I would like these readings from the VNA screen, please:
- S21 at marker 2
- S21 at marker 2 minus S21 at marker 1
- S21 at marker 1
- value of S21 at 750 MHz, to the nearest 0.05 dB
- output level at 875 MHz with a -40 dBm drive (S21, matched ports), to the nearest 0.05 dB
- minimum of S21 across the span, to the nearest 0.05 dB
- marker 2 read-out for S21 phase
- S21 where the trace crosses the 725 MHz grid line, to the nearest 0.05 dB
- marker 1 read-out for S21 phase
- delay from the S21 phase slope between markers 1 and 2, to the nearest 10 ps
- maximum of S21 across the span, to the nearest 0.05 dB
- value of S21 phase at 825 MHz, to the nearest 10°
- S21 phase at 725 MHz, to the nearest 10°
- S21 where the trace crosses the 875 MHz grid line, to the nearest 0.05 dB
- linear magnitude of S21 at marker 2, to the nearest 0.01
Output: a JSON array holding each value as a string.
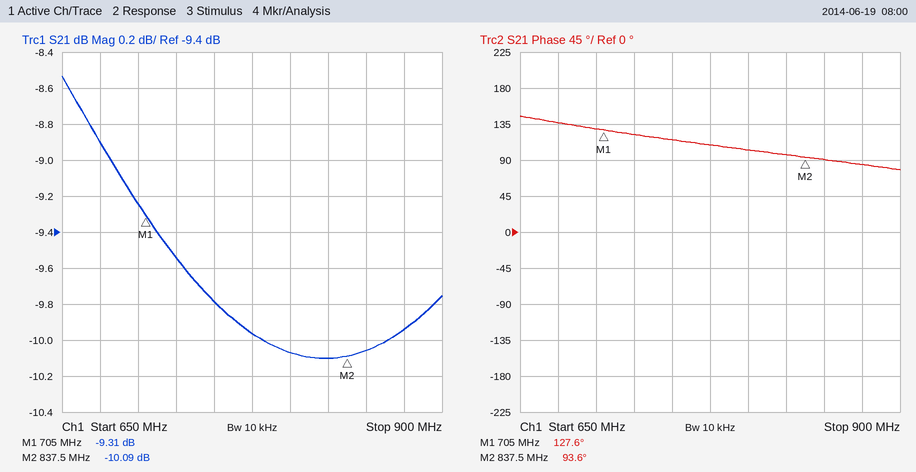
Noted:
["-10.09 dB", "-0.78 dB", "-9.31 dB", "-9.80 dB", "-49.95 dBm", "-10.10 dB", "93.6°", "-9.55 dB", "127.6°", "710 ps", "-8.55 dB", "100°", "120°", "-9.95 dB", "0.31"]
